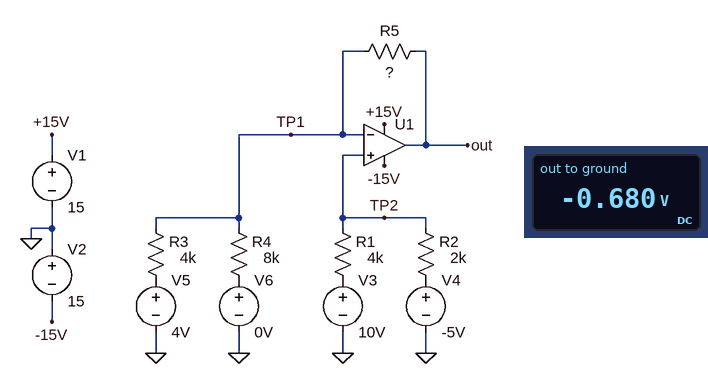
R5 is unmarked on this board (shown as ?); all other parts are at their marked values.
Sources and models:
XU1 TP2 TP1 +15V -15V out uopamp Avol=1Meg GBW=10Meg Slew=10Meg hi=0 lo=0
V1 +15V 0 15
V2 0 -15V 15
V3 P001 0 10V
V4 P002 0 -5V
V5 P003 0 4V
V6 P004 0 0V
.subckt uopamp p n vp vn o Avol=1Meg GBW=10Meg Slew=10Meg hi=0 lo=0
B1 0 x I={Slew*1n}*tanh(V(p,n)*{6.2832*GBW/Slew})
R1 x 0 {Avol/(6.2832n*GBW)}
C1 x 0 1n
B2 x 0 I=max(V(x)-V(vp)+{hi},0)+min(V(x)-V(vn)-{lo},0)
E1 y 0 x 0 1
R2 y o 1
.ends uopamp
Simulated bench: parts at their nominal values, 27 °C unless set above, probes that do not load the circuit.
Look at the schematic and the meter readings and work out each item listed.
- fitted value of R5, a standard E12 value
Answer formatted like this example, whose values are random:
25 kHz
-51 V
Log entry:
680 Ω
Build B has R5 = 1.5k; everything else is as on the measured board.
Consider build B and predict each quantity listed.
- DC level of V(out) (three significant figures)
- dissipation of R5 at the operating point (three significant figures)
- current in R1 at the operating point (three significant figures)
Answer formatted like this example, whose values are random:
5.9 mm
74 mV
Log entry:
-1.50 V
1.50 mW
2.50 mA
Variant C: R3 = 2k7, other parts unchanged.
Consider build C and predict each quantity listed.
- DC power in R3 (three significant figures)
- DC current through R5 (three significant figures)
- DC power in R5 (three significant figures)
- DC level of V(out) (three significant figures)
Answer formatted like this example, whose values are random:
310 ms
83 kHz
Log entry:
5.93 mW
1.48 mA
1.49 mW
-1.01 V
